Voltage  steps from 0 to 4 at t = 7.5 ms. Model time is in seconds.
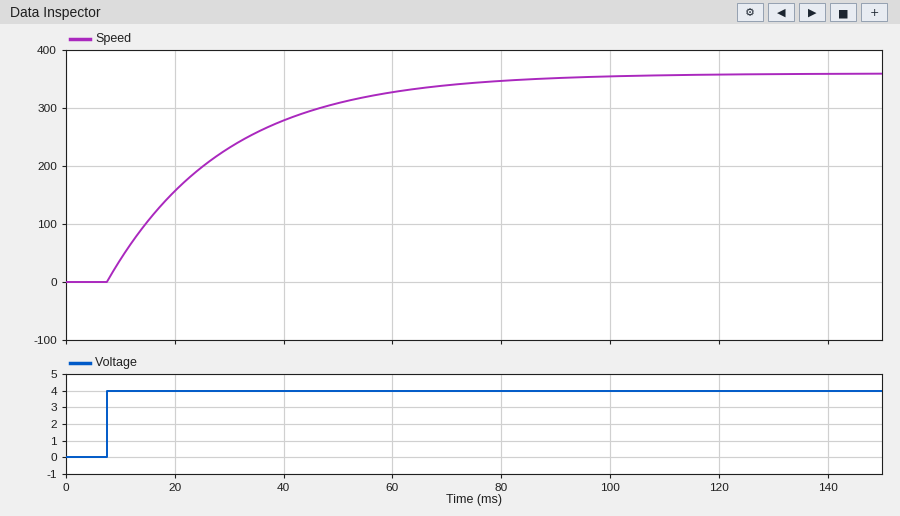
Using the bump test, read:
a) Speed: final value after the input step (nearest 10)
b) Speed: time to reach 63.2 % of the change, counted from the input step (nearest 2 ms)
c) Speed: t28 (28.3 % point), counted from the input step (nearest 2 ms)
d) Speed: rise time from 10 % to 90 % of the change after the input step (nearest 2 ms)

360
22 ms
8 ms
48 ms
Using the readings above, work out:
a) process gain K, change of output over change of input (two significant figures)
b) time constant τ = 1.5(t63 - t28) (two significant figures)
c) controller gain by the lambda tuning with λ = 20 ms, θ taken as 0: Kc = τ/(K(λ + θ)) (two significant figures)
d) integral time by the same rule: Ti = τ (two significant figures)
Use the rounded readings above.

90
21 ms
0.012
21 ms
